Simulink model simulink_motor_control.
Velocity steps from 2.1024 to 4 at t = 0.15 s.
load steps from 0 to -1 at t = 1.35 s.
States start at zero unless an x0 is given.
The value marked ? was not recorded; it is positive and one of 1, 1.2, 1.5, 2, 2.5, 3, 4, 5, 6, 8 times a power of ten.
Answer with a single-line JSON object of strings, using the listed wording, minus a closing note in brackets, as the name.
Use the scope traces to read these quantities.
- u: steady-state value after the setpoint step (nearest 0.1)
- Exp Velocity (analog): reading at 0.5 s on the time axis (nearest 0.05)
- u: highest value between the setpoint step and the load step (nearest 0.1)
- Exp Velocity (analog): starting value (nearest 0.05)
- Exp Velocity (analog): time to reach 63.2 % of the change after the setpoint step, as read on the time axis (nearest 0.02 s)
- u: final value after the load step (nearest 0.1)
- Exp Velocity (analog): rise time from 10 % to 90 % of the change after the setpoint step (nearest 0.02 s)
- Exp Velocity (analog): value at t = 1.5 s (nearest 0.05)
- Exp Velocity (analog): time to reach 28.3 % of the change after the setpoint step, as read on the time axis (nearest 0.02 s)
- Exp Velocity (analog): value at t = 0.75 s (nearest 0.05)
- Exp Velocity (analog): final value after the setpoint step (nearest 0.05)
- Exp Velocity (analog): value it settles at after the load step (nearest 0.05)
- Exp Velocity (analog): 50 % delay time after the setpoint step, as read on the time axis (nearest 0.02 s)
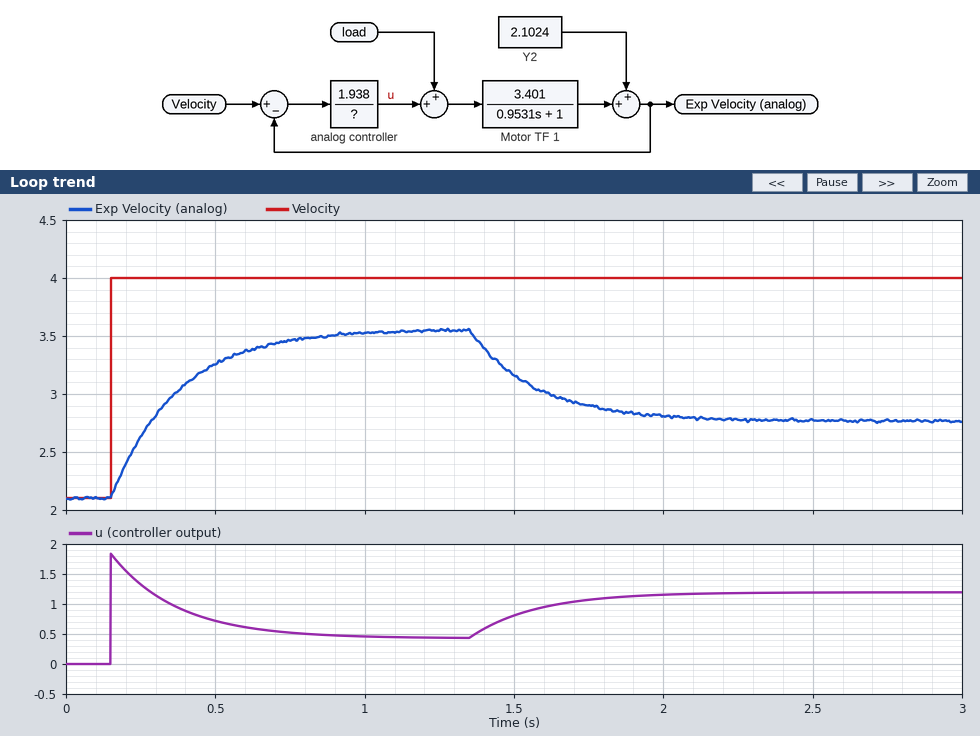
{"u: steady-state value after the setpoint step": "0.4", "Exp Velocity (analog): reading at 0.5 s on the time axis": "3.25", "u: highest value between the setpoint step and the load step": "1.8", "Exp Velocity (analog): starting value": "2.10", "Exp Velocity (analog): time to reach 63.2 % of the change after the setpoint step, as read on the time axis": "0.38 s", "u: final value after the load step": "1.2", "Exp Velocity (analog): rise time from 10 % to 90 % of the change after the setpoint step": "0.48 s", "Exp Velocity (analog): value at t = 1.5 s": "3.15", "Exp Velocity (analog): time to reach 28.3 % of the change after the setpoint step, as read on the time axis": "0.22 s", "Exp Velocity (analog): value at t = 0.75 s": "3.45", "Exp Velocity (analog): final value after the setpoint step": "3.55", "Exp Velocity (analog): value it settles at after the load step": "2.75", "Exp Velocity (analog): 50 % delay time after the setpoint step, as read on the time axis": "0.30 s"}
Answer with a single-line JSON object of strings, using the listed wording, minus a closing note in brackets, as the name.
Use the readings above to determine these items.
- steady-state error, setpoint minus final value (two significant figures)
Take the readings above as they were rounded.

{"steady-state error, setpoint minus final value": "0.45"}
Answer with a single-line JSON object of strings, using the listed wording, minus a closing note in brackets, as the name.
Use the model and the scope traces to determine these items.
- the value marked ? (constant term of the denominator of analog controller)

{"the value marked ?": "2"}
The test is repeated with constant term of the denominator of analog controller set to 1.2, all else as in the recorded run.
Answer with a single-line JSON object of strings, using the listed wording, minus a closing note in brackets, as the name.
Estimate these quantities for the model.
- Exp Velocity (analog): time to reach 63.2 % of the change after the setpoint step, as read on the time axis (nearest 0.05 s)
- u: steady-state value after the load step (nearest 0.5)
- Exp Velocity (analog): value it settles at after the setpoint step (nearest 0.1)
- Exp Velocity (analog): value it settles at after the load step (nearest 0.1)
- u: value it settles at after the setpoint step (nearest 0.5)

{"Exp Velocity (analog): time to reach 63.2 % of the change after the setpoint step, as read on the time axis": "0.30 s", "u: steady-state value after the load step": "1.5", "Exp Velocity (analog): value it settles at after the setpoint step": "3.7", "Exp Velocity (analog): value it settles at after the load step": "3.2", "u: value it settles at after the setpoint step": "0.5"}
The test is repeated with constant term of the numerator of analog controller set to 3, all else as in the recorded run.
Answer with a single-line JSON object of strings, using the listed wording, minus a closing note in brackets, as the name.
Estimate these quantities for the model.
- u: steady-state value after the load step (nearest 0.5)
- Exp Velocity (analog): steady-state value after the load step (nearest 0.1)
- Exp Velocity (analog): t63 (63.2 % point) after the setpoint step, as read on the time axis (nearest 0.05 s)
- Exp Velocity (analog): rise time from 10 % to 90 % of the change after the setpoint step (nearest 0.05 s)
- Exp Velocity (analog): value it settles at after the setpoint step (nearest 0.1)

{"u: steady-state value after the load step": "1.5", "Exp Velocity (analog): steady-state value after the load step": "3.1", "Exp Velocity (analog): t63 (63.2 % point) after the setpoint step, as read on the time axis": "0.30 s", "Exp Velocity (analog): rise time from 10 % to 90 % of the change after the setpoint step": "0.35 s", "Exp Velocity (analog): value it settles at after the setpoint step": "3.7"}
